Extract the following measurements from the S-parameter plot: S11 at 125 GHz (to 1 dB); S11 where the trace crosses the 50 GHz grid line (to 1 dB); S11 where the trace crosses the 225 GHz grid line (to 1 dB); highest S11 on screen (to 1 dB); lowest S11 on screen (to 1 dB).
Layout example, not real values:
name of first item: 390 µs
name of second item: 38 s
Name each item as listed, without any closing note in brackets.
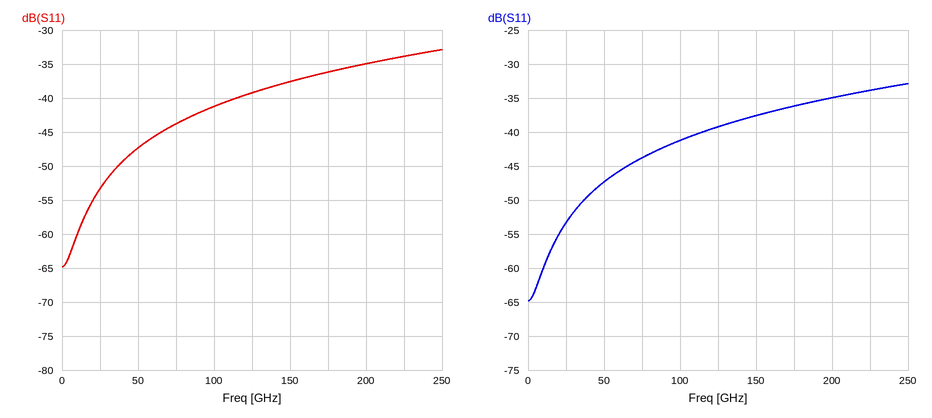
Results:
S11 at 125 GHz: -39 dB
S11 where the trace crosses the 50 GHz grid line: -47 dB
S11 where the trace crosses the 225 GHz grid line: -34 dB
highest S11 on screen: -33 dB
lowest S11 on screen: -65 dB
